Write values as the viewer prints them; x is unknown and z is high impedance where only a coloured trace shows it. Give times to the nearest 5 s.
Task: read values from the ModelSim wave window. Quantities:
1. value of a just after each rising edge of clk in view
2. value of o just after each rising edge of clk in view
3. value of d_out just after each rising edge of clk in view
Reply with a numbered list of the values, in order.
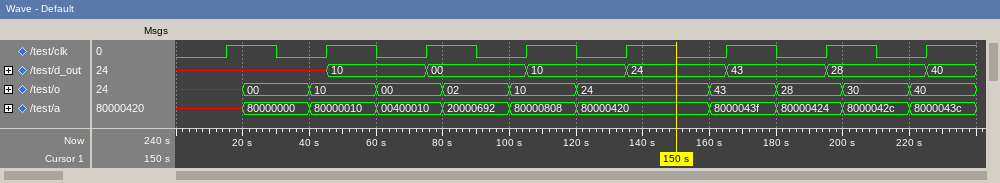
1. x, 80000010, 00400010, 80000808, 80000420, 8000043f, 80000424, 8000043c
2. x, 10, 00, 10, 24, 43, 28, 40
3. x, 10, 00, 10, 24, 43, 28, 40
